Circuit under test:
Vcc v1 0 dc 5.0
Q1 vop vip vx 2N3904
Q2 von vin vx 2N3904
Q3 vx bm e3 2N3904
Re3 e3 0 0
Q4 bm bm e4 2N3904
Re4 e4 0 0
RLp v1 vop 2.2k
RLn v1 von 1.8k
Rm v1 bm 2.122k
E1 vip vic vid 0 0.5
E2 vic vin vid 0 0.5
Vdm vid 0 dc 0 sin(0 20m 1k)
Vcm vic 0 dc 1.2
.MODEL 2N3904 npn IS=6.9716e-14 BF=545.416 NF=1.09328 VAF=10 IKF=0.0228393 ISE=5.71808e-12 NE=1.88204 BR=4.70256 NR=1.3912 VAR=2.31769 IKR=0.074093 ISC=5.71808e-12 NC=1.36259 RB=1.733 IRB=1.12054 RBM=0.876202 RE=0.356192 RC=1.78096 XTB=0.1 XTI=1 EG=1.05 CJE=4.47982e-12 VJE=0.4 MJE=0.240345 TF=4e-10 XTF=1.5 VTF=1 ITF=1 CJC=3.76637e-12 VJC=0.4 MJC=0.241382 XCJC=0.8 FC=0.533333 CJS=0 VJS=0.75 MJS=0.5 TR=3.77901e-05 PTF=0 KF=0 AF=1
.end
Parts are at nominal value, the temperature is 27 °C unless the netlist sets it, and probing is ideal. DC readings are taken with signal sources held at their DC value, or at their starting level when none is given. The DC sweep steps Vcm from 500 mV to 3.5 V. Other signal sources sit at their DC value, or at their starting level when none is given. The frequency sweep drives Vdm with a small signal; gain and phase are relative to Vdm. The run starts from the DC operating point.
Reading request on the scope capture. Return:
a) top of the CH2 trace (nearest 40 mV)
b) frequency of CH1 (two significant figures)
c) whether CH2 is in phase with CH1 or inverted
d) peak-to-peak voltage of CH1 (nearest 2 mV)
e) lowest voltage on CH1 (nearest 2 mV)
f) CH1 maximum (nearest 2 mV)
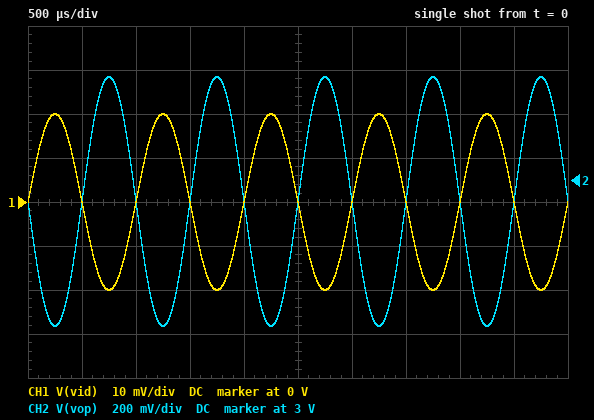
3.48 V
1.0 kHz
inverted
40 mV
-20 mV
20 mV
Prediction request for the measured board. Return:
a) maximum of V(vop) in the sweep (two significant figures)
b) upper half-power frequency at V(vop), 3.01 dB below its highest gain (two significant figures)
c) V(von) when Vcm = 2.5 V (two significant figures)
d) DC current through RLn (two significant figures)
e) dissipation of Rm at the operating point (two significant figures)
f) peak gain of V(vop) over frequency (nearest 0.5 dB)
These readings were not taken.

5.0 V
33 MHz
2.9 V
990 µA
8.7 mW
29.0 dB
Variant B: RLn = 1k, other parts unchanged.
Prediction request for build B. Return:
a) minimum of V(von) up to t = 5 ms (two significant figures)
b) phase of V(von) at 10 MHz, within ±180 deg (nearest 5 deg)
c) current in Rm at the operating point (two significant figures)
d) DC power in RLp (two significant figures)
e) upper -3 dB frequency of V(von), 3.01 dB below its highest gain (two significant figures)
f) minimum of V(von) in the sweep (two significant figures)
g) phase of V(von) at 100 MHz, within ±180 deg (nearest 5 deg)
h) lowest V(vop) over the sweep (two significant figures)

3.7 V
-5 deg
2.0 mA
1.9 mW
83 MHz
3.6 V
-55 deg
2.5 V
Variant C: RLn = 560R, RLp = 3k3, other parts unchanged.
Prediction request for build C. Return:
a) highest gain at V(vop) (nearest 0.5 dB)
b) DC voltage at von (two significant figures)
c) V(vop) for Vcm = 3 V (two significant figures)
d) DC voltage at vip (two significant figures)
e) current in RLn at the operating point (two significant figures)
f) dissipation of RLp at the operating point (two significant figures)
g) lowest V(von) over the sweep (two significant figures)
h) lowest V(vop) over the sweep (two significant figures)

32.5 dB
4.4 V
2.4 V
1.2 V
1.1 mA
2.4 mW
4.2 V
1.9 V
